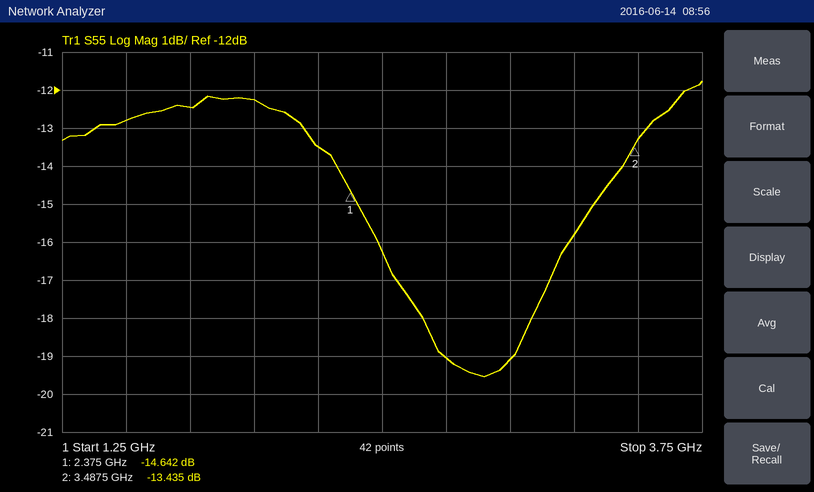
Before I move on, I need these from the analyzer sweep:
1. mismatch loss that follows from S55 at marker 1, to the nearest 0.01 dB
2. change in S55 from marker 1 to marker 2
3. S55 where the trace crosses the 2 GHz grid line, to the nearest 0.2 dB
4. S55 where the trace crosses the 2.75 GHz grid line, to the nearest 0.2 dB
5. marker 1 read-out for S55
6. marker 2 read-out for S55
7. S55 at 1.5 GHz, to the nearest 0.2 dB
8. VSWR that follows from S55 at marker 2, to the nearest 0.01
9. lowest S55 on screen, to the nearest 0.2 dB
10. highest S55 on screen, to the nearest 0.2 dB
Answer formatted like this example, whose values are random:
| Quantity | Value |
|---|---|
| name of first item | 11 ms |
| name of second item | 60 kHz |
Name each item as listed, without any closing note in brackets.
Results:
| Quantity | Value |
|---|---|
| mismatch loss that follows from S55 at marker 1, to the nearest 0.01 dB | 0.15 dB |
| change in S55 from marker 1 to marker 2 | 1.207 dB |
| S55 where the trace crosses the 2 GHz grid line, to the nearest 0.2 dB | -12.2 dB |
| S55 where the trace crosses the 2.75 GHz grid line, to the nearest 0.2 dB | -19.0 dB |
| marker 1 read-out for S55 | -14.642 dB |
| marker 2 read-out for S55 | -13.435 dB |
| S55 at 1.5 GHz, to the nearest 0.2 dB | -12.8 dB |
| VSWR that follows from S55 at marker 2, to the nearest 0.01 | 1.54 |
| lowest S55 on screen, to the nearest 0.2 dB | -19.6 dB |
| highest S55 on screen, to the nearest 0.2 dB | -11.8 dB |
